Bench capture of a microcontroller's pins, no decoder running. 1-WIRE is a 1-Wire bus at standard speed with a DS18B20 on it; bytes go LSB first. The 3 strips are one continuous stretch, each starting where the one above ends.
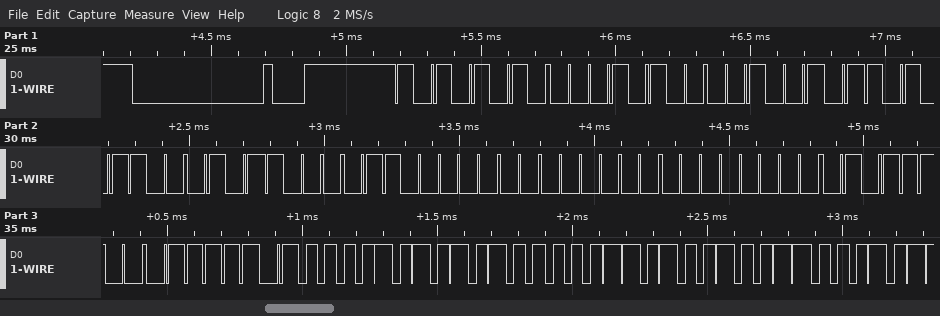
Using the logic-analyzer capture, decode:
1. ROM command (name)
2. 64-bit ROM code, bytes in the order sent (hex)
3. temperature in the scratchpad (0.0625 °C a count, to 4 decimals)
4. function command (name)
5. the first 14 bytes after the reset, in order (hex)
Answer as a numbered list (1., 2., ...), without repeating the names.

1. Match ROM
2. 28 A4 35 1A 06 00 00 3A
3. 85.0000 °C
4. Read Scratchpad
5. 55 28 A4 35 1A 06 00 00 3A BE 50 05 4B 46
